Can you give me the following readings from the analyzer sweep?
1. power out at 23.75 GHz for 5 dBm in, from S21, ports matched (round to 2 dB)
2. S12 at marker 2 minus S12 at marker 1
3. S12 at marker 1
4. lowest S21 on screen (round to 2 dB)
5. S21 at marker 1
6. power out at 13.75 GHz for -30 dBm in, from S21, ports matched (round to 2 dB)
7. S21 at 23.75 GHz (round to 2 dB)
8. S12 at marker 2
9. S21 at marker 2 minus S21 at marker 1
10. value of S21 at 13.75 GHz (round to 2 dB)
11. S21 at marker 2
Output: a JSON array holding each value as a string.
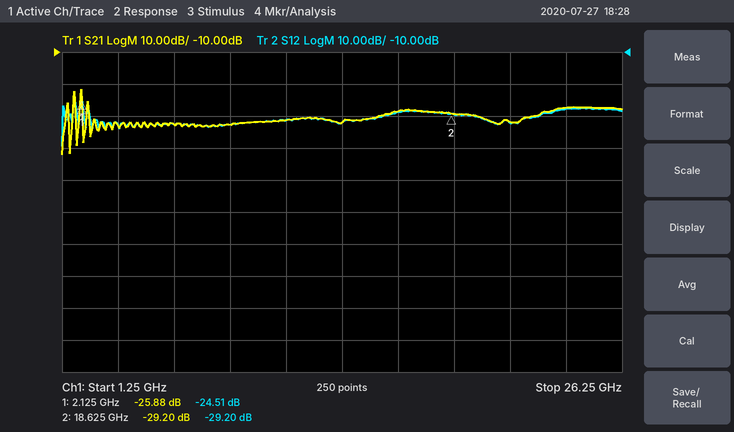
["-22 dBm", "-4.69 dB", "-24.51 dB", "-42 dB", "-25.88 dB", "-62 dBm", "-28 dB", "-29.20 dB", "-3.32 dB", "-32 dB", "-29.20 dB"]
